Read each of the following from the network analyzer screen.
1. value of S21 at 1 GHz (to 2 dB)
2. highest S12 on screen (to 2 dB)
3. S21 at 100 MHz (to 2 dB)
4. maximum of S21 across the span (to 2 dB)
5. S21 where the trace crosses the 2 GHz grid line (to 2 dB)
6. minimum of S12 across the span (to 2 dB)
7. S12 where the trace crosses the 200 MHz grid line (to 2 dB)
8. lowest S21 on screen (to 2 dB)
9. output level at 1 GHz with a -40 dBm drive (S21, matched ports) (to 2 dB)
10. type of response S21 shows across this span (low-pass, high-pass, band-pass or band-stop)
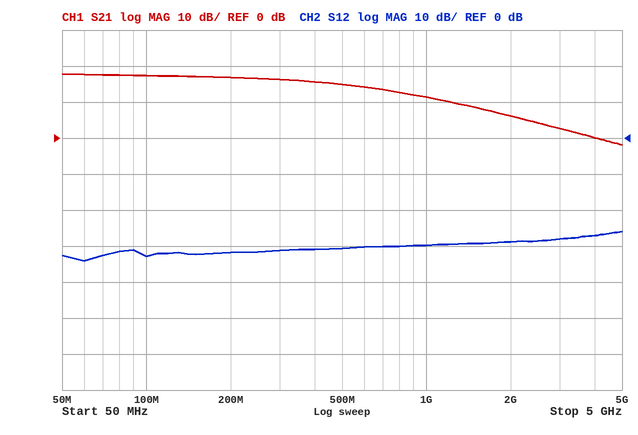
12 dB
-26 dB
18 dB
18 dB
6 dB
-34 dB
-32 dB
-2 dB
-28 dBm
low-pass
